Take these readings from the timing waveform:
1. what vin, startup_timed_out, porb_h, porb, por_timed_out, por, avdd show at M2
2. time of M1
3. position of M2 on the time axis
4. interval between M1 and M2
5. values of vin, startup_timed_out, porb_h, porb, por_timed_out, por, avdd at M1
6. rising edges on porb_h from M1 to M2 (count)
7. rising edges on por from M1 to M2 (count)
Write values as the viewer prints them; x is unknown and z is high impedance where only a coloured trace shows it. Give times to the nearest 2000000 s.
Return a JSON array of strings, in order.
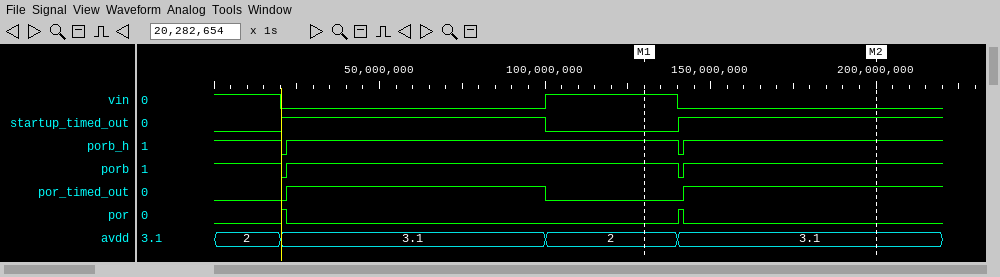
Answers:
["vin=0, startup_timed_out=1, porb_h=1, porb=1, por_timed_out=1, por=0, avdd=3.1", "130000000 s", "200000000 s", "70000000 s", "vin=1, startup_timed_out=0, porb_h=1, porb=1, por_timed_out=0, por=0, avdd=2", "1", "1"]
